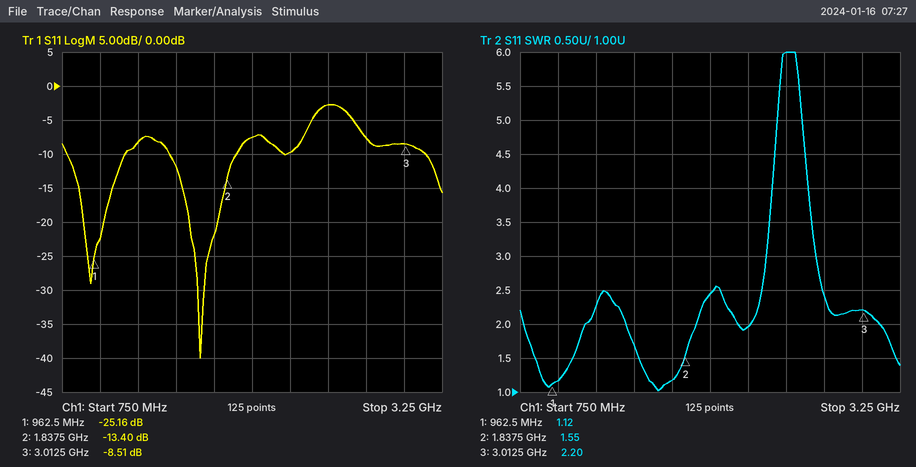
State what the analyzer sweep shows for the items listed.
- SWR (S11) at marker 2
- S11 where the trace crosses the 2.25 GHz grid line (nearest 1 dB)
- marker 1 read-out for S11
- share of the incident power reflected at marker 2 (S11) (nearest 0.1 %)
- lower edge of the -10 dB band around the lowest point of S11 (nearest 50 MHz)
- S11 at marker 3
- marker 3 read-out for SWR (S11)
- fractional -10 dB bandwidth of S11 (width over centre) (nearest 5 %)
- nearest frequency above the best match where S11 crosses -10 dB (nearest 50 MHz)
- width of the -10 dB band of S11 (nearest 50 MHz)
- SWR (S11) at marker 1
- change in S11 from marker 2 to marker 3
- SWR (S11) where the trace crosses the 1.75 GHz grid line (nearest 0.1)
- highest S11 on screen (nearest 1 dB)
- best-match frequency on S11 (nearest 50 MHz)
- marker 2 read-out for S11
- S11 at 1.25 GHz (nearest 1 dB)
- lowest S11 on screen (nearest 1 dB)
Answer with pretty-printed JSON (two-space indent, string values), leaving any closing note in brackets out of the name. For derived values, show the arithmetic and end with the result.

{
  "SWR (S11) at marker 2": "1.55",
  "S11 where the trace crosses the 2.25 GHz grid line": "-10 dB",
  "marker 1 read-out for S11": "-25.16 dB",
  "share of the incident power reflected at marker 2 (S11)": "10^(-13.4/10) ≈ 4.6 %",
  "lower edge of the -10 dB band around the lowest point of S11": "1.45 GHz",
  "S11 at marker 3": "-8.51 dB",
  "marker 3 read-out for SWR": "2.20",
  "fractional -10 dB bandwidth of S11 (width over centre)": "450 MHz / 1.675 GHz ≈ 26.9 %, so 25 % to the nearest 5 %",
  "nearest frequency above the best match where S11 crosses -10 dB": "1.90 GHz",
  "width of the -10 dB band of S11": "1.90 GHz − 1.45 GHz = 450 MHz",
  "SWR (S11) at marker 1": "1.12",
  "change in S11 from marker 2 to marker 3": "-8.51 − (-13.4) = 4.89 dB",
  "SWR (S11) where the trace crosses the 1.75 GHz grid line": "1.2",
  "highest S11 on screen": "-3 dB",
  "best-match frequency on S11": "1.65 GHz",
  "marker 2 read-out for S11": "-13.40 dB",
  "S11 at 1.25 GHz": "-8 dB",
  "lowest S11 on screen": "-40 dB"
}
